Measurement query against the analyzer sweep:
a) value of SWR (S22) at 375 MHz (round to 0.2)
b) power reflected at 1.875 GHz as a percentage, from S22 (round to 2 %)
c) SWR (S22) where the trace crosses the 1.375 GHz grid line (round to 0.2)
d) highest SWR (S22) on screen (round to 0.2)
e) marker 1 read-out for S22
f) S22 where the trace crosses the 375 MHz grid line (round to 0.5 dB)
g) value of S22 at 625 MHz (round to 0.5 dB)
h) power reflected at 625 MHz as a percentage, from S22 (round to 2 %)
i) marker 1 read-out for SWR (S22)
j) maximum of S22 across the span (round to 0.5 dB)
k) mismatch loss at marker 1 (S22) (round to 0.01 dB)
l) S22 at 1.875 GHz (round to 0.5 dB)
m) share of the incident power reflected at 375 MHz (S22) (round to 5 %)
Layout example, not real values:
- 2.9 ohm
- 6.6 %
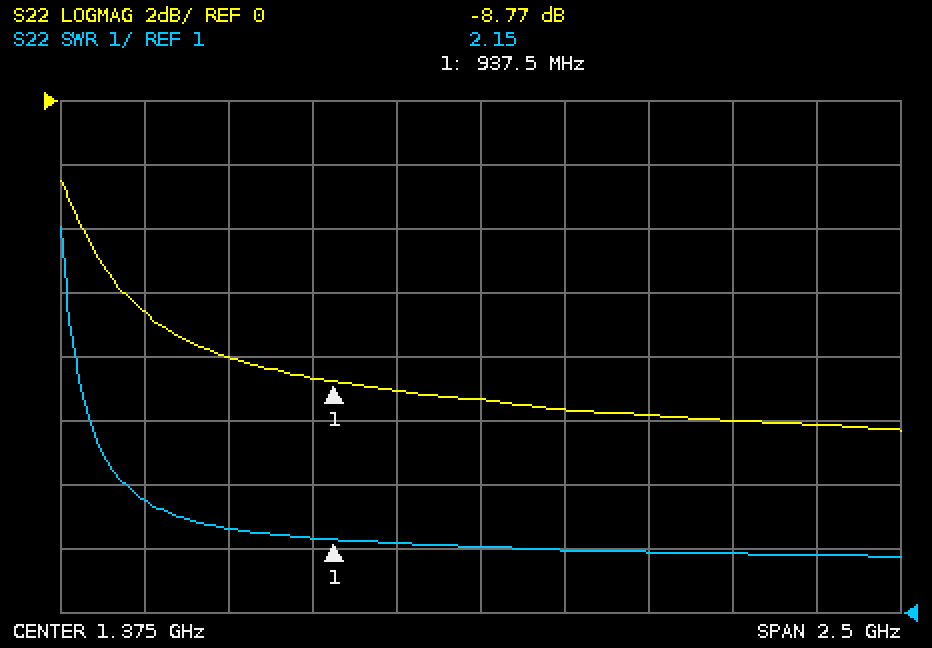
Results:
- 2.8
- 10 %
- 2.0
- 7.0
- -8.77 dB
- -6.5 dB
- -8.0 dB
- 16 %
- 2.15
- -2.5 dB
- 0.62 dB
- -10.0 dB
- 20 %
